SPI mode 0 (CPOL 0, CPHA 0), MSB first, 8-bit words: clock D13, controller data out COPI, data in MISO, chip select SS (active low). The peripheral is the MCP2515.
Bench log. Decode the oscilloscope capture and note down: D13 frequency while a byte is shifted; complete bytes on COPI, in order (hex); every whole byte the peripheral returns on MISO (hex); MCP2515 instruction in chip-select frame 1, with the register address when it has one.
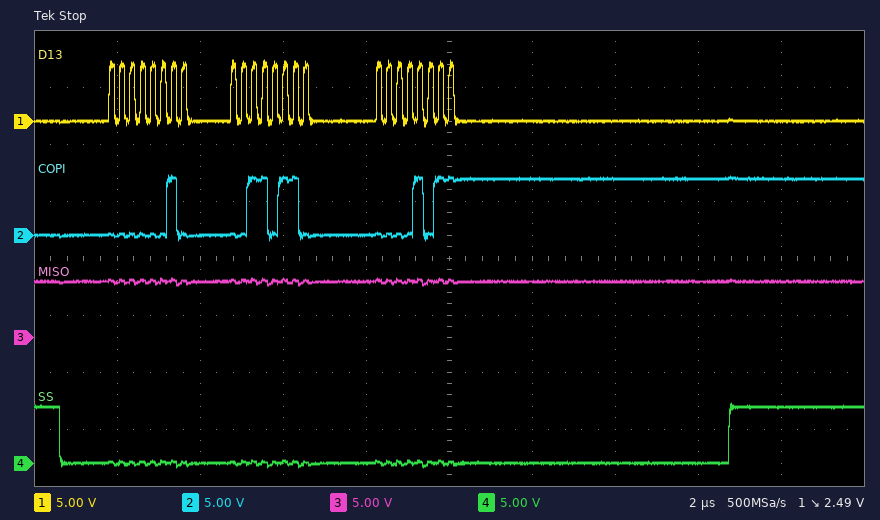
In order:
4 MHz
02 36 0B
FF FF FF
WRITE 0x36
